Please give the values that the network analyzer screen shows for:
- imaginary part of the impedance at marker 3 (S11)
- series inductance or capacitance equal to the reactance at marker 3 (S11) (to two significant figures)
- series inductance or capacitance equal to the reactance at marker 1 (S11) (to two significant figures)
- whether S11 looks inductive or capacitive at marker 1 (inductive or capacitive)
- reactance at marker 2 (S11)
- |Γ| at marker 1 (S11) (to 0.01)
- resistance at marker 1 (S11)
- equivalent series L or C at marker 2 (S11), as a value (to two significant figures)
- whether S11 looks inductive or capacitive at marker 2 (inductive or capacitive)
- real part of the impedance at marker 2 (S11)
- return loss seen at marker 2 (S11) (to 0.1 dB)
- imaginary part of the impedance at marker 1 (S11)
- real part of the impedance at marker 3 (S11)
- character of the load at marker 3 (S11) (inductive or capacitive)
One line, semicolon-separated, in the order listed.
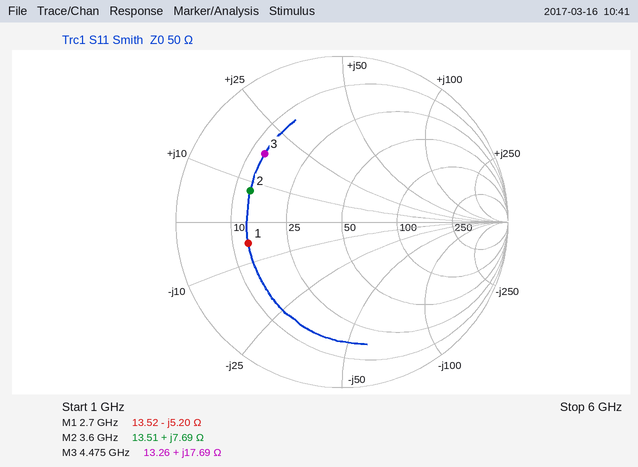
+17.69 Ω; 630 pH; 11 pF; capacitive; +7.69 Ω; 0.58; 13.52 Ω; 340 pH; inductive; 13.51 Ω; 4.7 dB; -5.20 Ω; 13.26 Ω; inductive
